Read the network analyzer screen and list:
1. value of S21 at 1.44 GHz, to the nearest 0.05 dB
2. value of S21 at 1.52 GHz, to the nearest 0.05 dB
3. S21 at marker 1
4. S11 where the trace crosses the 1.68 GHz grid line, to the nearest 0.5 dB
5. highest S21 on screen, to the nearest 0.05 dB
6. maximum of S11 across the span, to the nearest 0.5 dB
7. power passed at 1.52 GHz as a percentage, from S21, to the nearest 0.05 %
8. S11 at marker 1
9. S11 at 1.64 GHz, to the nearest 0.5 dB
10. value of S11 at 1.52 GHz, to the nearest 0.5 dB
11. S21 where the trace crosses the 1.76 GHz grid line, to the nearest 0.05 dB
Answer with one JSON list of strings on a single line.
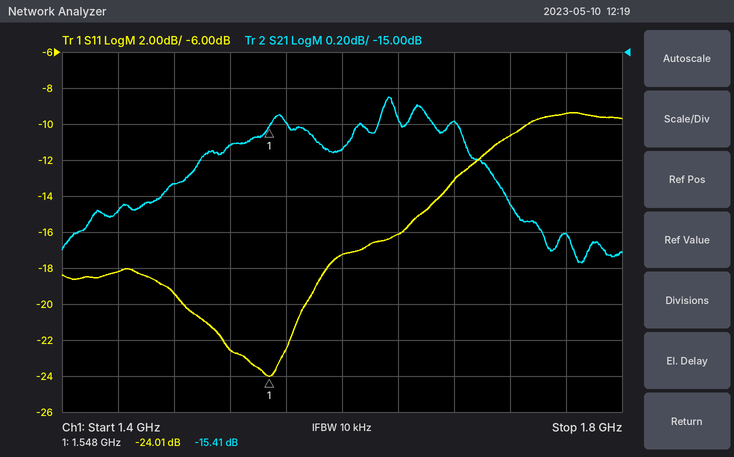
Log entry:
["-15.90 dB", "-15.50 dB", "-15.41 dB", "-13.0 dB", "-15.25 dB", "-9.5 dB", "2.80 %", "-24.01 dB", "-16.0 dB", "-22.5 dB", "-16.00 dB"]
